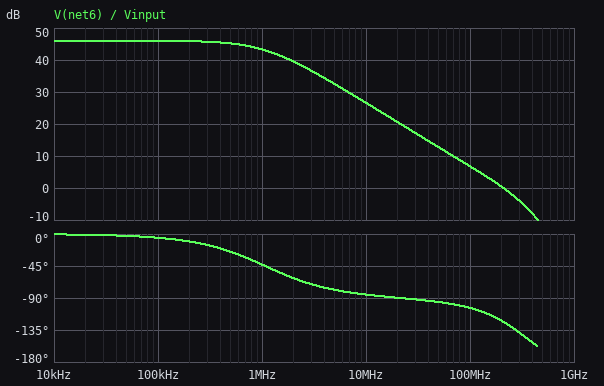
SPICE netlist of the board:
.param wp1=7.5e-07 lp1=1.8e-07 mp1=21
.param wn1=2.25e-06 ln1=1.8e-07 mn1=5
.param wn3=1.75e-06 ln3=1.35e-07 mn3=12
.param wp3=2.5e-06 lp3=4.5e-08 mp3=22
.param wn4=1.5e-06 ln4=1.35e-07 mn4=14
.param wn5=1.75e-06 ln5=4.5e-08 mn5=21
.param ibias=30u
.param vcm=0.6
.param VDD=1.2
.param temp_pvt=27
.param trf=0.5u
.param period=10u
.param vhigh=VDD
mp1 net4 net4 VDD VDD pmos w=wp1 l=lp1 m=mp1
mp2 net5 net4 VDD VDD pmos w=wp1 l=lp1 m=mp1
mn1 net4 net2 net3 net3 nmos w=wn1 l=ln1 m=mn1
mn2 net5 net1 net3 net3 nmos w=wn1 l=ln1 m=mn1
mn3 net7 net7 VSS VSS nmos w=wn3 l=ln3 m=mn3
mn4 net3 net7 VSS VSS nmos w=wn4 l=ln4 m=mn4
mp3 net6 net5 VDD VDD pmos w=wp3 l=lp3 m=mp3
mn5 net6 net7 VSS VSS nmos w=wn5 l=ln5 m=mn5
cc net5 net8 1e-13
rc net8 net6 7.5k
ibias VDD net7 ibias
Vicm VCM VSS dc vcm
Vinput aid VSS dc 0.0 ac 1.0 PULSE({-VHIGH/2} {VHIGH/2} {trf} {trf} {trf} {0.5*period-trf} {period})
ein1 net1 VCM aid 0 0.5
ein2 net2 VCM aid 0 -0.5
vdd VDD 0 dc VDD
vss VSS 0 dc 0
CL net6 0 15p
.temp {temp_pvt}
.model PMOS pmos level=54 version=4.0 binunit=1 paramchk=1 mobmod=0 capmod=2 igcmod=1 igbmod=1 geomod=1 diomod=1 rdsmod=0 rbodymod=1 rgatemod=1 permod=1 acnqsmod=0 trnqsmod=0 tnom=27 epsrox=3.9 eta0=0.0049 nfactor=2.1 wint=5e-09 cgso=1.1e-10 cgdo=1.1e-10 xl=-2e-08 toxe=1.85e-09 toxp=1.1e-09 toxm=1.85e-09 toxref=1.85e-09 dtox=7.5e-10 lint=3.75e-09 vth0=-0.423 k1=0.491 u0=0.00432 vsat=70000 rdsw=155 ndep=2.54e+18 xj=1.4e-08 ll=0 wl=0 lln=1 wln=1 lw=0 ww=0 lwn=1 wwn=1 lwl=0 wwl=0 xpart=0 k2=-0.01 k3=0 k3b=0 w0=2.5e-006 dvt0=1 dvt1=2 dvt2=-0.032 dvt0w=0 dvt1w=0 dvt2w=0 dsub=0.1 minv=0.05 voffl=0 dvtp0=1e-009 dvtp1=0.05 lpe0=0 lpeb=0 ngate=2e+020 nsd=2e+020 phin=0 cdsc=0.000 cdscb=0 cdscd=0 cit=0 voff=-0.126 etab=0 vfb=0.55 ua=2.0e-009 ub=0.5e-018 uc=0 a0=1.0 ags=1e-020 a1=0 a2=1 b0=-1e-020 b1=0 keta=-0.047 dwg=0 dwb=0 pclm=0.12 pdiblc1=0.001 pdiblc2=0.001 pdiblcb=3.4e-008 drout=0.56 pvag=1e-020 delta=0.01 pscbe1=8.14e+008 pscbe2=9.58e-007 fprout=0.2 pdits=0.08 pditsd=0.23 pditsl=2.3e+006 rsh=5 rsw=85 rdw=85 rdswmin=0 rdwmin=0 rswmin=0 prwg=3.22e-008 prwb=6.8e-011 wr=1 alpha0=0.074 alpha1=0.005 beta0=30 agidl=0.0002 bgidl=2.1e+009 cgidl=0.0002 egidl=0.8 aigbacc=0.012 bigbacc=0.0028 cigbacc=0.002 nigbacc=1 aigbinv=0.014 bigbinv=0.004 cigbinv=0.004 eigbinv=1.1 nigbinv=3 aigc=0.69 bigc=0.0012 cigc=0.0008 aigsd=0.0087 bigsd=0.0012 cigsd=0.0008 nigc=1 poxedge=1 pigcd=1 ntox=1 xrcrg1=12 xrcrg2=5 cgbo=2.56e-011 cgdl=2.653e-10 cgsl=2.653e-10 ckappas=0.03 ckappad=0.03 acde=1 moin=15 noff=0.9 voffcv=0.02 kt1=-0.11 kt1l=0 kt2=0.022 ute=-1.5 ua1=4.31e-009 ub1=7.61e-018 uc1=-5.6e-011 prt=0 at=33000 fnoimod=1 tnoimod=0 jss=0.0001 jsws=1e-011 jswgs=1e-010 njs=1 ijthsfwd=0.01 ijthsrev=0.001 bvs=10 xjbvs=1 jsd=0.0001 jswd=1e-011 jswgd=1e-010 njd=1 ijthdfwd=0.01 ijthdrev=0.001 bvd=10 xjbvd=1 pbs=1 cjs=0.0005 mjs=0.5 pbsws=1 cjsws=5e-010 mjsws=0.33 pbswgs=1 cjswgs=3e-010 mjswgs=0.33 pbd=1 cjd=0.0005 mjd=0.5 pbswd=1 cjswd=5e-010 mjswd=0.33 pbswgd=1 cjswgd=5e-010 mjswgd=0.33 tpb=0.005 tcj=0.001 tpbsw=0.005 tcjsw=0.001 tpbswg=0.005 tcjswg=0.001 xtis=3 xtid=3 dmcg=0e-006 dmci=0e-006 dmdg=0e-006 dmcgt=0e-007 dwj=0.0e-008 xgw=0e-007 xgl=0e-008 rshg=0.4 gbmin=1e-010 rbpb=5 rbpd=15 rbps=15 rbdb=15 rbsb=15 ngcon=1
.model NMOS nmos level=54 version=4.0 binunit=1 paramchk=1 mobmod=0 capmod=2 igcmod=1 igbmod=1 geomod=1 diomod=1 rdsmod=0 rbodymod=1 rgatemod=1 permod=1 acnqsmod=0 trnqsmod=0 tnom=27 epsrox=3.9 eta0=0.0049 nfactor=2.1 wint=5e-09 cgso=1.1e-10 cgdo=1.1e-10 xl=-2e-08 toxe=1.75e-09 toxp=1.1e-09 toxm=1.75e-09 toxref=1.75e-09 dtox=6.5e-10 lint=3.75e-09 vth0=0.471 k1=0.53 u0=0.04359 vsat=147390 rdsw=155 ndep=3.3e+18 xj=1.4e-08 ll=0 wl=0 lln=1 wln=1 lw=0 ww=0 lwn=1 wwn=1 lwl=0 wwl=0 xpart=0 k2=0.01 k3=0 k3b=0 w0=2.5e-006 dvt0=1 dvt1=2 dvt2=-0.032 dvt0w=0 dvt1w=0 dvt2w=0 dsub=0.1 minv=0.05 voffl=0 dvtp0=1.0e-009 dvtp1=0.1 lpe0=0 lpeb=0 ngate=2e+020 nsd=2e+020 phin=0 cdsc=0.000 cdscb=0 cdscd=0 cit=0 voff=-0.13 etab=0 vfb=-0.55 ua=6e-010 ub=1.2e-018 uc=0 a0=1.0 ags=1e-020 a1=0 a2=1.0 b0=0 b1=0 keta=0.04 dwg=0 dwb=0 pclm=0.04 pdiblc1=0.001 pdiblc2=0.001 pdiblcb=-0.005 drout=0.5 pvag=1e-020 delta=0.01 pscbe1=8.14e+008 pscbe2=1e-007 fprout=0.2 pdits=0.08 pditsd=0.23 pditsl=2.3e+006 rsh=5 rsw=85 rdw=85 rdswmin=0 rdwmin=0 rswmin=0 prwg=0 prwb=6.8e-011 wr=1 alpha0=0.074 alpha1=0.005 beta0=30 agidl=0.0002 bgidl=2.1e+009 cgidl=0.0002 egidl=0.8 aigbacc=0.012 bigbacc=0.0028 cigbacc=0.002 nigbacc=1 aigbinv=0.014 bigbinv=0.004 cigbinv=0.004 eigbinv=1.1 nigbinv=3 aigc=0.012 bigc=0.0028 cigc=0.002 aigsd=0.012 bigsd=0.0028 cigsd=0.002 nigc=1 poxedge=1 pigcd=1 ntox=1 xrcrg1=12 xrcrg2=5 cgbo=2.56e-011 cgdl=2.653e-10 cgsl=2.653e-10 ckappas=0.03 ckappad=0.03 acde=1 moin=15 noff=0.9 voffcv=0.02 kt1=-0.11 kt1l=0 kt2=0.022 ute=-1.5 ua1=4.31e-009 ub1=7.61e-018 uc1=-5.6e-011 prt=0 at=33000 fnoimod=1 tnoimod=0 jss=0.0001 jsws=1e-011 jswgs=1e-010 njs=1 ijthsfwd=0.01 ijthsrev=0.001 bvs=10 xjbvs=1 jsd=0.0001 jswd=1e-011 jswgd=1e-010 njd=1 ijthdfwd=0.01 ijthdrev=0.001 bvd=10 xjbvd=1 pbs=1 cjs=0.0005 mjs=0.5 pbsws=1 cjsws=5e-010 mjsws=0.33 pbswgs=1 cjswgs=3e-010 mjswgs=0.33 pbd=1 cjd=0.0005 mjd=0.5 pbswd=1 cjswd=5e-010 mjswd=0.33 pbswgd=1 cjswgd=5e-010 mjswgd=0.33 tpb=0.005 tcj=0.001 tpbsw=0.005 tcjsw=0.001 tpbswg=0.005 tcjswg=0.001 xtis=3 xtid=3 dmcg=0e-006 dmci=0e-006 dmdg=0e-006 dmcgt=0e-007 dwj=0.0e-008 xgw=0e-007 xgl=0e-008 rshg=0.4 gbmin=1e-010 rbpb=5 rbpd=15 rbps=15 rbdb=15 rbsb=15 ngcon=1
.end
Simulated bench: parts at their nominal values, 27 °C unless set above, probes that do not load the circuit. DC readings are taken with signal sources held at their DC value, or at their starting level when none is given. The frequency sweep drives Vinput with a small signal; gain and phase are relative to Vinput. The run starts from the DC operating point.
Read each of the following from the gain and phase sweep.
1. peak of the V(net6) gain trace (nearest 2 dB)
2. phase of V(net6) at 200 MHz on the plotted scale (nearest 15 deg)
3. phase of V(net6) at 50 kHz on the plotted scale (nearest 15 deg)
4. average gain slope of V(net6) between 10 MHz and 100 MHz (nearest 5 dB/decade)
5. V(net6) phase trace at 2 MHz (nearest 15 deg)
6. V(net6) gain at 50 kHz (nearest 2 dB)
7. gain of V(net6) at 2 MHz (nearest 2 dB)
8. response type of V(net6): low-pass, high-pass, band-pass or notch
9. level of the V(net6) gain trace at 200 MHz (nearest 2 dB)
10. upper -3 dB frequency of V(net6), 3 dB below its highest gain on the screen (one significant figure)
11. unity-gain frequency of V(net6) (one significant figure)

46 dB
-120 deg
0 deg
-20 dB/decade
-60 deg
46 dB
40 dB
low-pass
0 dB
1 MHz
200 MHz
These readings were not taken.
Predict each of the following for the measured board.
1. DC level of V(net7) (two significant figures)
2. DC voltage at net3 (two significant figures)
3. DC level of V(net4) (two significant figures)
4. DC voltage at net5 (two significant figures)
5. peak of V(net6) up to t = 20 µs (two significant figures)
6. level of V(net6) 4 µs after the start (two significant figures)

380 mV
210 mV
730 mV
730 mV
1.1 V
1.1 V
